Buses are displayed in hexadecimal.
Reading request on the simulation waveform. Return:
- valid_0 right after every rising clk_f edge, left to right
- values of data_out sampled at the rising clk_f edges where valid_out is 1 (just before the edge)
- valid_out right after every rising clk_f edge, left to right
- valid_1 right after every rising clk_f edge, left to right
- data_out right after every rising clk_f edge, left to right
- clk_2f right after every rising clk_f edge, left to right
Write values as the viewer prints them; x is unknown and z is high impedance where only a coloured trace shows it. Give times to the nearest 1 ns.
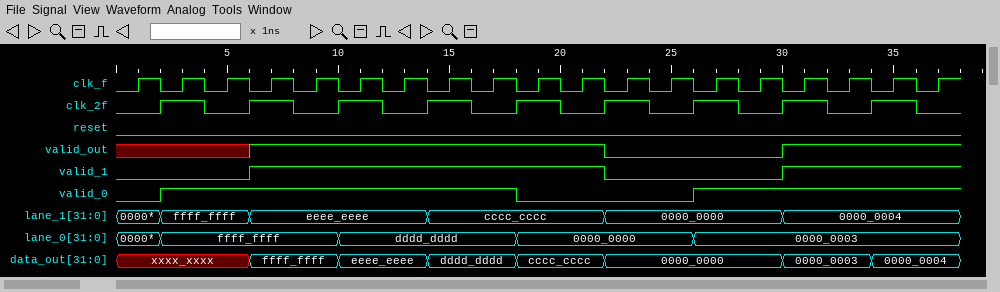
0 1 1 1 1 1 1 1 1 0 0 0 0 1 1 1 1 1 1
ffff_ffff, ffff_ffff, eeee_eeee, eeee_eeee, dddd_dddd, dddd_dddd, cccc_cccc, cccc_cccc, 0000_0003, 0000_0003, 0000_0004, 0000_0004
x x x 1 1 1 1 1 1 1 1 0 0 0 0 1 1 1 1
0 0 0 1 1 1 1 1 1 1 1 0 0 0 0 1 1 1 1
xxxx_xxxx, xxxx_xxxx, xxxx_xxxx, ffff_ffff, ffff_ffff, eeee_eeee, eeee_eeee, dddd_dddd, dddd_dddd, cccc_cccc, cccc_cccc, 0000_0000, 0000_0000, 0000_0000, 0000_0000, 0000_0003, 0000_0003, 0000_0004, 0000_0004
0 1 0 1 0 1 0 1 0 1 0 1 0 1 0 1 0 1 0
